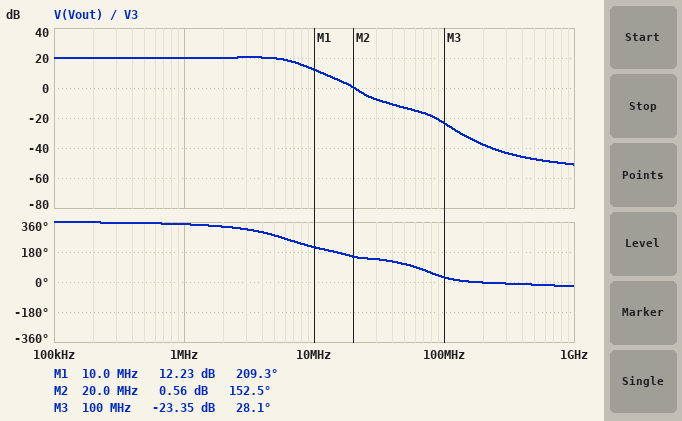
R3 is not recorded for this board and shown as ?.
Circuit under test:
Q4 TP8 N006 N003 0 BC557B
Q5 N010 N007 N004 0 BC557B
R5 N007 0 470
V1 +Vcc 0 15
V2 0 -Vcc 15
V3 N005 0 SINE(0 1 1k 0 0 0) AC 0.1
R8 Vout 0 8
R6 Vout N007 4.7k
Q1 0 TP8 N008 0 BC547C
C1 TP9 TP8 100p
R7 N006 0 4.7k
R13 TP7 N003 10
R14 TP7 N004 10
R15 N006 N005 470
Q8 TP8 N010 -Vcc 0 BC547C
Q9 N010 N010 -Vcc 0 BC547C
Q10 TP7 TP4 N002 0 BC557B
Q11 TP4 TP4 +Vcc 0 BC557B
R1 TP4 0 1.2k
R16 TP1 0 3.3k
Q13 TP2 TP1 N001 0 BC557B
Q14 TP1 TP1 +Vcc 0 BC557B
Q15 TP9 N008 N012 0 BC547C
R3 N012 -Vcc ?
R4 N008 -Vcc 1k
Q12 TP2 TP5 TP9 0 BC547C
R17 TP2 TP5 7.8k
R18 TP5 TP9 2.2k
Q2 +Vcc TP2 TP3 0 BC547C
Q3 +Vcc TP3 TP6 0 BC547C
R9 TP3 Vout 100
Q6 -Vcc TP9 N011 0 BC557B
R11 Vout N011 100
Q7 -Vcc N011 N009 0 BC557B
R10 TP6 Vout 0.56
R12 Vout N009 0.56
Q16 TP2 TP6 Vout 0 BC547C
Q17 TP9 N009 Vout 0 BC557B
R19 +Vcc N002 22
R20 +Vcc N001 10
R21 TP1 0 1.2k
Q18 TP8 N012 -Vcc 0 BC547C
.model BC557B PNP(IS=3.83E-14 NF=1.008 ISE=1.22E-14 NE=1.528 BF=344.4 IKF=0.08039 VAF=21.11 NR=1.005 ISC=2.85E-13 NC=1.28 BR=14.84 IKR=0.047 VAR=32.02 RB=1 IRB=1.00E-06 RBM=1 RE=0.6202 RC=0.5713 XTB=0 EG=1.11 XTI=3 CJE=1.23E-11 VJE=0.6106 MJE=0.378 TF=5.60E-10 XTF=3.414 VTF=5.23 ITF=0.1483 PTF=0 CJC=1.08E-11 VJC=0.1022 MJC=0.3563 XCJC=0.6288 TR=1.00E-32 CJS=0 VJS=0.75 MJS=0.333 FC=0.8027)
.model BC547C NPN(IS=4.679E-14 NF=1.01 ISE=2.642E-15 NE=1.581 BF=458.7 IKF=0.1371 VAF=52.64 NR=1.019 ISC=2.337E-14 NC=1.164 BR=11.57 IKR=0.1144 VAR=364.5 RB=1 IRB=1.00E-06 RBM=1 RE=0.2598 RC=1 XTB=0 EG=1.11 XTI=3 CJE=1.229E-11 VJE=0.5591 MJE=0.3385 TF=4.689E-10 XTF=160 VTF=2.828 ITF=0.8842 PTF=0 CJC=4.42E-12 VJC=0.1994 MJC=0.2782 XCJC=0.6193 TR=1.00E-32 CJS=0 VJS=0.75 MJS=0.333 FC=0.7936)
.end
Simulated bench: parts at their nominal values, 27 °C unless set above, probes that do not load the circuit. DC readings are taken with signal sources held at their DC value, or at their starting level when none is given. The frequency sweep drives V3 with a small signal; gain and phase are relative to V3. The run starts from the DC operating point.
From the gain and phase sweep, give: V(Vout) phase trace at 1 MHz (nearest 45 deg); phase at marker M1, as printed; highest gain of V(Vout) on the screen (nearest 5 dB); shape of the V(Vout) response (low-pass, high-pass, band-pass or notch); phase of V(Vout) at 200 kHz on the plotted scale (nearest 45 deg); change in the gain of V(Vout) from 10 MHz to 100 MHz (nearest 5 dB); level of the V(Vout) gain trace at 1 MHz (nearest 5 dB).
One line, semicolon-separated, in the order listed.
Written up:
360 deg; 209.3 deg; 20 dB; low-pass; 360 deg; -35 dB; 20 dB
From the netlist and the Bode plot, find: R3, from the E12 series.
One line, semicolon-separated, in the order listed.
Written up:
22 Ω
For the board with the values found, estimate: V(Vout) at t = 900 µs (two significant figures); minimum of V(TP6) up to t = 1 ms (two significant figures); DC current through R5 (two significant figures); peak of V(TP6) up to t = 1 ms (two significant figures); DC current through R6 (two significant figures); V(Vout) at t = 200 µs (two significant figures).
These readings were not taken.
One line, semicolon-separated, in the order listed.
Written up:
-5.9 V; -10 V; 4.5 µA; 10 V; 2.0 µA; 9.5 V
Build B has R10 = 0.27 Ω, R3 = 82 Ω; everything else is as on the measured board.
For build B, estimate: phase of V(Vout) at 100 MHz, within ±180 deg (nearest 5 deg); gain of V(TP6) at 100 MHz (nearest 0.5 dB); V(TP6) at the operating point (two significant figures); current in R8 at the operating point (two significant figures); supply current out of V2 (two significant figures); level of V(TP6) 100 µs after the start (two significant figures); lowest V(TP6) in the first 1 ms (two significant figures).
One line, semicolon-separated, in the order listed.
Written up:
0 deg; -26.0 dB; 54 mV; 2.2 mA; 150 mA; 6.1 V; -9.3 V
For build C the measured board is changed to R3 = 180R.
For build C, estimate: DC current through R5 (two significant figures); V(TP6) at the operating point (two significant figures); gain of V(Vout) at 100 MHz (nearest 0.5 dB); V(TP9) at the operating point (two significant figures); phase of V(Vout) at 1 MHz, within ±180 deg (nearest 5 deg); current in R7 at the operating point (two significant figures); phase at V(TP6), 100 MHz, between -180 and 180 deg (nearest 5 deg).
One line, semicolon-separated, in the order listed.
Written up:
1.7 mA; 9.6 V; -66.5 dB; 8.5 V; 35 deg; 470 nA; -120 deg
